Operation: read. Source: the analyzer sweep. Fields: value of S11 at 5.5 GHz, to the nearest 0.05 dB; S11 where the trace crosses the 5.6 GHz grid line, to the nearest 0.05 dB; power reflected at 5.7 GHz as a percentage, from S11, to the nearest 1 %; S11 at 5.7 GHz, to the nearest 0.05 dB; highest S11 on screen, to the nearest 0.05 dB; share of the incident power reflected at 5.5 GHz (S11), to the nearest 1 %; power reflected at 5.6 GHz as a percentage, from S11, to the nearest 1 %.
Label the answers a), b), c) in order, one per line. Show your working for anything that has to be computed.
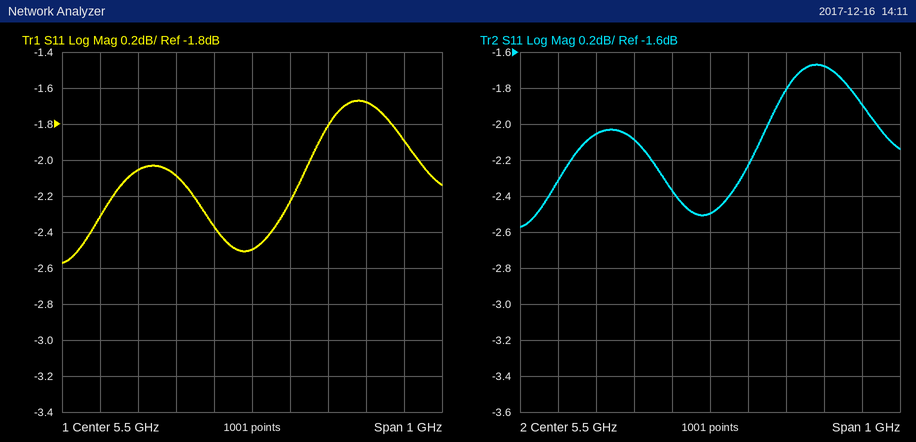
a) -2.50 dB
b) -2.25 dB
c) 10^(-1.8/10) ≈ 66 %
d) -1.80 dB
e) -1.65 dB
f) 10^(-2.5/10) ≈ 56 %
g) 10^(-2.25/10) ≈ 60 %
